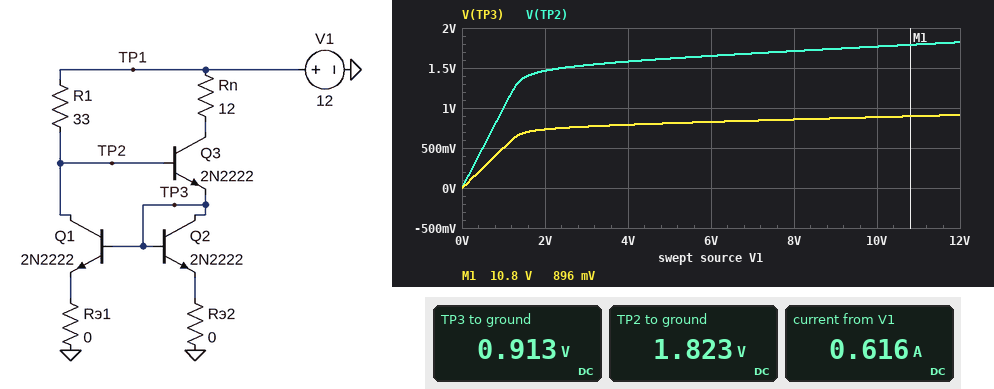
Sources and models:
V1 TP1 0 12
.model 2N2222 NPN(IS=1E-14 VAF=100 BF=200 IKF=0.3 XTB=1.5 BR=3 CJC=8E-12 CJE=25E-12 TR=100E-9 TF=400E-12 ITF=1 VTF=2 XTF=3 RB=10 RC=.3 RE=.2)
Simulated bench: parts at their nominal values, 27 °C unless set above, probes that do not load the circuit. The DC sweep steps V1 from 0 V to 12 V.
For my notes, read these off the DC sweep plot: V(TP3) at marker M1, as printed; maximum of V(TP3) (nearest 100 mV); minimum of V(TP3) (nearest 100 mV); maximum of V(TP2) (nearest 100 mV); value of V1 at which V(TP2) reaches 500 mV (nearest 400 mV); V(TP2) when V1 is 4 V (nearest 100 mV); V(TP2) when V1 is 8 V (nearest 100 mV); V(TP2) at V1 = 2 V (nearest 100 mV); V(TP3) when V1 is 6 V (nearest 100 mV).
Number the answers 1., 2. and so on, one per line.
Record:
1. 896 mV
2. 900 mV
3. 0 V
4. 1.8 V
5. 400 mV
6. 1.6 V
7. 1.7 V
8. 1.5 V
9. 800 mV
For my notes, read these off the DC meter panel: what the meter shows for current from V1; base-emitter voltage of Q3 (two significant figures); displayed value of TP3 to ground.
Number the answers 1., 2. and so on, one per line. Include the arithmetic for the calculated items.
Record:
1. 0.616 A
2. 1.823 V - 913 mV = 910 mV
3. 0.913 V
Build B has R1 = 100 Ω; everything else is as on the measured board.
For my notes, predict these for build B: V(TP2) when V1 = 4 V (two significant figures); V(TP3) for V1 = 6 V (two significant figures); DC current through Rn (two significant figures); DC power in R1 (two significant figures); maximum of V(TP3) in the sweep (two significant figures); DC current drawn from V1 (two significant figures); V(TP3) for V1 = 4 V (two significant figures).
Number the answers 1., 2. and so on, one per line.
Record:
1. 1.5 V
2. 770 mV
3. 100 mA
4. 1.1 W
5. 810 mV
6. 210 mA
7. 750 mV
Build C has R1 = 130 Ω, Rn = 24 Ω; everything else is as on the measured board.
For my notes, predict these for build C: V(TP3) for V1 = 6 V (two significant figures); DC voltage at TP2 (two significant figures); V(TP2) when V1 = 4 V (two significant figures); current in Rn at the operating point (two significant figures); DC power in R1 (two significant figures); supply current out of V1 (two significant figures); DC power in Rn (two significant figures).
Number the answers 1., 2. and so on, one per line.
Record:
1. 760 mV
2. 1.6 V
3. 1.5 V
4. 80 mA
5. 830 mW
6. 160 mA
7. 150 mW
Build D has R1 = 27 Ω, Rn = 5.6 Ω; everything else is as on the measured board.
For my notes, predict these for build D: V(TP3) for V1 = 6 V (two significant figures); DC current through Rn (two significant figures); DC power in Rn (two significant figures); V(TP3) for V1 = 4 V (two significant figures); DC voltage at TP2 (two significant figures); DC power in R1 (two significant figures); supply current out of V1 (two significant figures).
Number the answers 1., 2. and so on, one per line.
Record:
1. 840 mV
2. 370 mA
3. 780 mW
4. 800 mV
5. 1.9 V
6. 3.8 W
7. 750 mA
